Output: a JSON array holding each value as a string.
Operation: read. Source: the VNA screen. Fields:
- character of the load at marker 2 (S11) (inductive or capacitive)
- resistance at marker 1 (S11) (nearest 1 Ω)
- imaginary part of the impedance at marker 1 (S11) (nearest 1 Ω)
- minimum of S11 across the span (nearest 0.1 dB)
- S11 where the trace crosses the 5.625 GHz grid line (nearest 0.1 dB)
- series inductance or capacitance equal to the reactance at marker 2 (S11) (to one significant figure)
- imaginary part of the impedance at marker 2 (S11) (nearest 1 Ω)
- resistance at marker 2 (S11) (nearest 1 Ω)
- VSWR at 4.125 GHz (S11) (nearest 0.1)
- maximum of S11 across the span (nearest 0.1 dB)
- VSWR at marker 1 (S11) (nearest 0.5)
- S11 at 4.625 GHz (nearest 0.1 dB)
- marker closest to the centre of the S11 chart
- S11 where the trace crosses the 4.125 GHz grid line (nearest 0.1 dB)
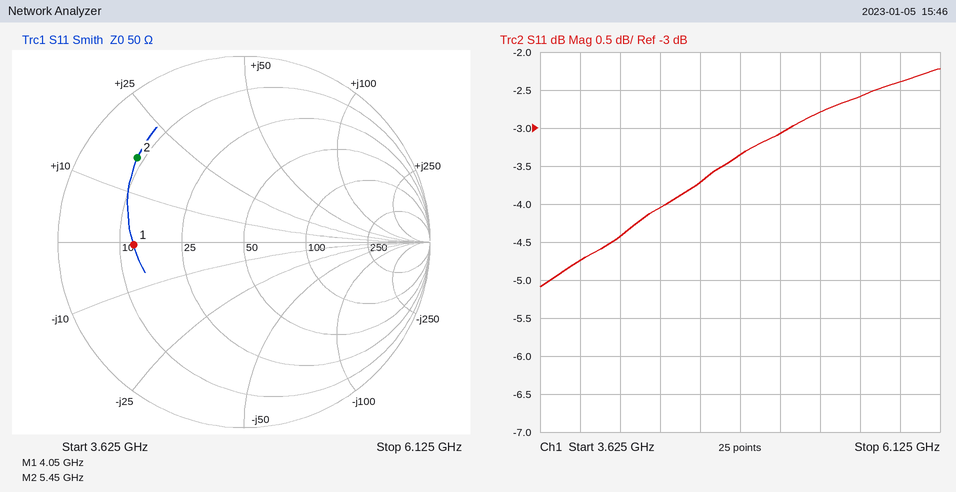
["inductive", "13 Ω", "-1 Ω", "-5.1 dB", "-2.6 dB", "500 pH", "+17 Ω", "9 Ω", "4.0", "-2.2 dB", "4.0", "-3.7 dB", "marker 1", "-4.4 dB"]
